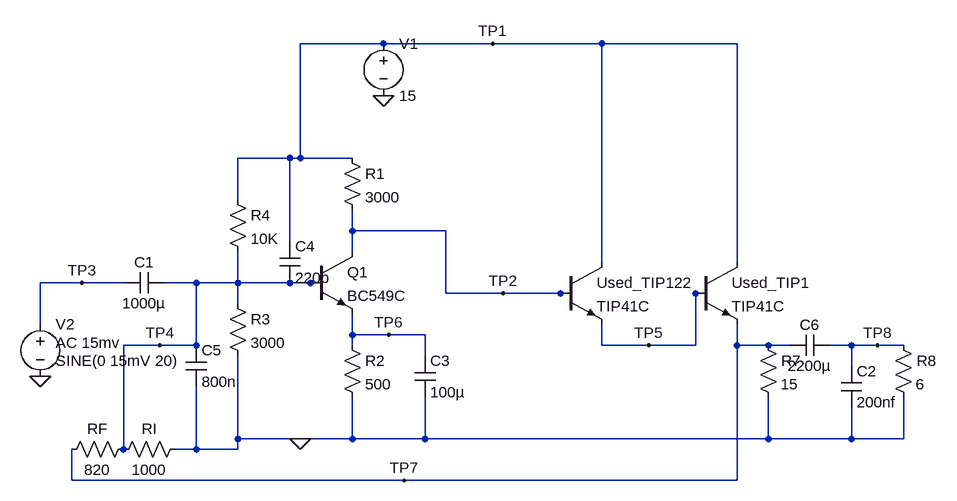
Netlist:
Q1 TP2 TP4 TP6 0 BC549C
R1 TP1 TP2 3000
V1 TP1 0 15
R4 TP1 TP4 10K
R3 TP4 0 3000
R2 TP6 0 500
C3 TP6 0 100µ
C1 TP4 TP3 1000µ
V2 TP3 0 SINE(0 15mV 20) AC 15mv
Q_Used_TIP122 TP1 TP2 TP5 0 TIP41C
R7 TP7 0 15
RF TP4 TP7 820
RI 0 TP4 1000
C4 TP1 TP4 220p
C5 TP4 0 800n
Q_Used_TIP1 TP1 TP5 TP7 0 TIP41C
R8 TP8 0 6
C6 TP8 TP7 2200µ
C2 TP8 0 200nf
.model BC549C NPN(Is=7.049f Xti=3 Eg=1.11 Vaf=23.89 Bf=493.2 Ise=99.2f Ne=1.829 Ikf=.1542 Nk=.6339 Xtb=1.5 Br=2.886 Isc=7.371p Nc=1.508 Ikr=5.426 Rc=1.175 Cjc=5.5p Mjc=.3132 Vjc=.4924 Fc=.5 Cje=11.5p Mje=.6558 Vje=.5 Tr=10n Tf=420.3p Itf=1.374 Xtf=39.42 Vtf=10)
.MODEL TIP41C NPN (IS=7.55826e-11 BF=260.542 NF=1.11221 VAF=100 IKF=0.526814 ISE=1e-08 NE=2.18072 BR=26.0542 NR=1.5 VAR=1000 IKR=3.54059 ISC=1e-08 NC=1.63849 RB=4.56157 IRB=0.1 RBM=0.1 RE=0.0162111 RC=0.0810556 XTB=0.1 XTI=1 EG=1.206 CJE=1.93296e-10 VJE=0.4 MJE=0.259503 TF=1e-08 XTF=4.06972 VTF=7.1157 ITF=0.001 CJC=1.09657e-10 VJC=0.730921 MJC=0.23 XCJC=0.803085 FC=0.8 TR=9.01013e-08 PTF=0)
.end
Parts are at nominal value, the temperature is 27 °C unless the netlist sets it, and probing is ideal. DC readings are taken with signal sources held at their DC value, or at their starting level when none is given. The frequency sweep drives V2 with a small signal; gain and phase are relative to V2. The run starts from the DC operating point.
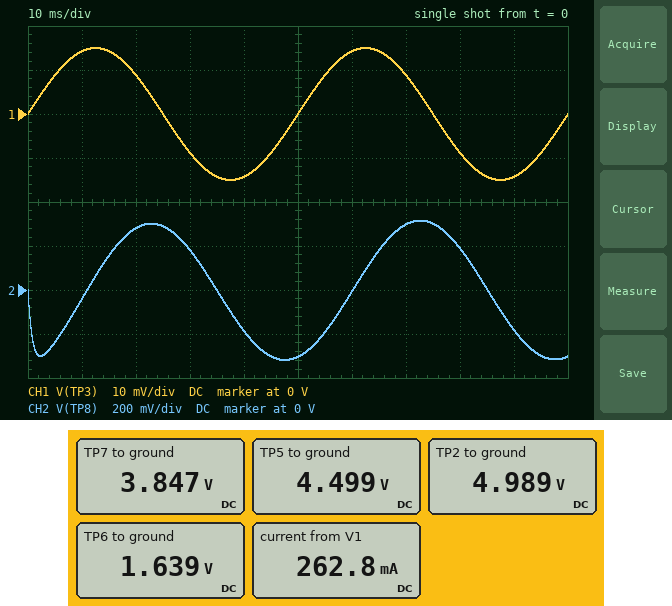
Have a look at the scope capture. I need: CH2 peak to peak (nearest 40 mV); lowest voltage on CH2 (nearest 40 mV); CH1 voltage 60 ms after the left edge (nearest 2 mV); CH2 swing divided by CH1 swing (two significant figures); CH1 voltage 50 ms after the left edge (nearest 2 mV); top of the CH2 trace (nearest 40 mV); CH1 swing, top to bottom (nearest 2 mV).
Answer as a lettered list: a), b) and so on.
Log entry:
a) 640 mV
b) -320 mV
c) 14 mV
d) 21
e) 0 V
f) 320 mV
g) 30 mV
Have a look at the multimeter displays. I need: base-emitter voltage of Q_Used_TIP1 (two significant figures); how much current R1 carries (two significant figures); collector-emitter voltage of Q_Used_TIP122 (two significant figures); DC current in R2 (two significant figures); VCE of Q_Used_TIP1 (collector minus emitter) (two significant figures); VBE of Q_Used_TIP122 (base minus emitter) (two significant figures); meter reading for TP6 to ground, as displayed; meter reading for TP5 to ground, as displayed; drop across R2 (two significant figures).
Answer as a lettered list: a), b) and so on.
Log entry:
a) 650 mV
b) 3.3 mA
c) 11 V
d) 3.3 mA
e) 11 V
f) 490 mV
g) 1.639 V
h) 4.499 V
i) 1.6 V
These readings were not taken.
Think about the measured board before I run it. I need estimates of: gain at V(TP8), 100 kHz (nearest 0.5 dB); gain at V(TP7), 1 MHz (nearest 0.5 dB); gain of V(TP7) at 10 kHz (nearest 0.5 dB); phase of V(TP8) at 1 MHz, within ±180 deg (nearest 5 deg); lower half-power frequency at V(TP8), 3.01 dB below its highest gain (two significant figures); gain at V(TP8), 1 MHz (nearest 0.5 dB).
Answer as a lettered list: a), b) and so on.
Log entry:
a) 49.0 dB
b) 11.0 dB
c) 47.5 dB
d) -50 deg
e) 160 kHz
f) 11.0 dB
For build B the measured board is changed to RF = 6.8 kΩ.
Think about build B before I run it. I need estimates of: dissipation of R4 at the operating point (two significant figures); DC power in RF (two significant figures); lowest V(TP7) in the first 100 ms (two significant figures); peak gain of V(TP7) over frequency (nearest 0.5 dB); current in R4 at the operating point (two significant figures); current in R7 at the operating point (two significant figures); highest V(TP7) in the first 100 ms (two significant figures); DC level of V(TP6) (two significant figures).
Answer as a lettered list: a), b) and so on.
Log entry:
a) 18 mW
b) 5.2 mW
c) 7.1 V
d) 52.0 dB
e) 1.3 mA
f) 510 mA
g) 8.1 V
h) 980 mV
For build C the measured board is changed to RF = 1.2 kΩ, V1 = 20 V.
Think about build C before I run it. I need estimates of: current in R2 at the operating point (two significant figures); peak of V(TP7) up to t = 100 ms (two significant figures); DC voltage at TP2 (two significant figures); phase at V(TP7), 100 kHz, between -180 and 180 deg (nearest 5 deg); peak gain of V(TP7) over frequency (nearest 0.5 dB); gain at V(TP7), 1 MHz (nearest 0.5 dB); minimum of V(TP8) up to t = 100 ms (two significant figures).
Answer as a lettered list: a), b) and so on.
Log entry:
a) 4.4 mA
b) 5.9 V
c) 6.6 V
d) 160 deg
e) 61.5 dB
f) 16.5 dB
g) -350 mV
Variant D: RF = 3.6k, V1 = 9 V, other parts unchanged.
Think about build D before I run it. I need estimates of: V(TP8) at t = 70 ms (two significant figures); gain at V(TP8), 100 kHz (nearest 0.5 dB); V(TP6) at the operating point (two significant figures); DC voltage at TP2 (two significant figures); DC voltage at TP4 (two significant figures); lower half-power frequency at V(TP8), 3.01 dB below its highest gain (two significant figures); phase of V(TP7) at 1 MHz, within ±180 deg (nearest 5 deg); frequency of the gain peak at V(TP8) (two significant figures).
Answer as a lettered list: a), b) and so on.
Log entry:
a) 300 mV
b) 43.0 dB
c) 560 mV
d) 5.4 V
e) 1.2 V
f) 90 kHz
g) -45 deg
h) 140 kHz
